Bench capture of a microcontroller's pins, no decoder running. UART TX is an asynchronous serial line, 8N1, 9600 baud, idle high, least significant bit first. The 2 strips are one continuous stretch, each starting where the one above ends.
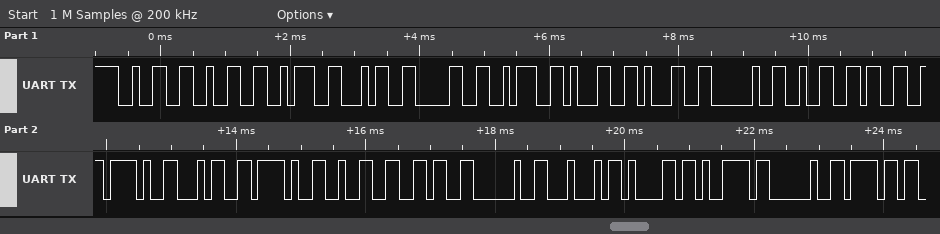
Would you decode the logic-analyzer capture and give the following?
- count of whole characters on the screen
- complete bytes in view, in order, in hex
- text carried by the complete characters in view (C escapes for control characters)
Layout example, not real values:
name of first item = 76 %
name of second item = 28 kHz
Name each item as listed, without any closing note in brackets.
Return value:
count of whole characters on the screen = 22
complete bytes in view, in order, in hex = 0x32 0x32 0x3A 0x34 0x30 0x3A 0x31 0x31 0x20 0x32 0x33 0x2F 0x34 0x2F 0x32 0x36 0x20 0x44 0x61 0x79 0x20 0x6F
text carried by the complete characters in view = "22:40:11 23/4/26 Day o"
